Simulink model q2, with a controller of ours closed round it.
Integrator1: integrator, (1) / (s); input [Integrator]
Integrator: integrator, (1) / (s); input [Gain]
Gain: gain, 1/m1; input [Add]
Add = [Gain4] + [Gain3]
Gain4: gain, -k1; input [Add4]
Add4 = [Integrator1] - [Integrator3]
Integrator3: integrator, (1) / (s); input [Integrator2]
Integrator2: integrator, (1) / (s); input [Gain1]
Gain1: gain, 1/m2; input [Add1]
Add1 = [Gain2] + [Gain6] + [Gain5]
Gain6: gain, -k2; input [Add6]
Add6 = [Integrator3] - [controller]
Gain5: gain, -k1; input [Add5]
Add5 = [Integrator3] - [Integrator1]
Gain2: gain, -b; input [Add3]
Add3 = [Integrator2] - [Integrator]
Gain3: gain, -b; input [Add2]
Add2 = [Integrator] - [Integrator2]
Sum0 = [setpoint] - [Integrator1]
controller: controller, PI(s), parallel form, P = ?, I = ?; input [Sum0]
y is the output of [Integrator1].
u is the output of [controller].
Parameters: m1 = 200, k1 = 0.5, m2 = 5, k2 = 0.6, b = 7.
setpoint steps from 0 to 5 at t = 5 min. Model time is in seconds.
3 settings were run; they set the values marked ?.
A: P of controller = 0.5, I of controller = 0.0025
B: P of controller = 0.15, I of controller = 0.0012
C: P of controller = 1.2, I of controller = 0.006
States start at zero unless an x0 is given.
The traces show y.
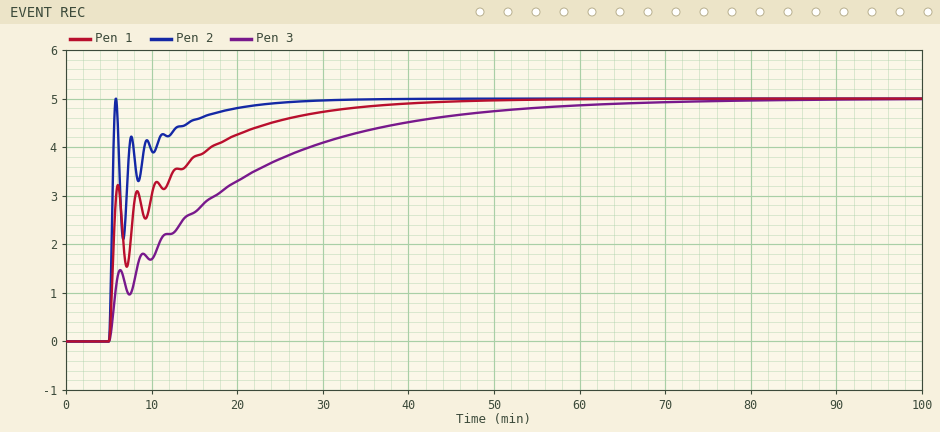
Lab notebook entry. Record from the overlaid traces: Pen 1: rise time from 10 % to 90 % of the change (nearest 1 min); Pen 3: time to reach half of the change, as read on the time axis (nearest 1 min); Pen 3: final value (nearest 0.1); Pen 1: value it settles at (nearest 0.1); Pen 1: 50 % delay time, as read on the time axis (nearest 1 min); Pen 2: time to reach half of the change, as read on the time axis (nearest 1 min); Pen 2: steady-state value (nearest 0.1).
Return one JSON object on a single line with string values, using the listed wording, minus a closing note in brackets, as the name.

{"Pen 1: rise time from 10 % to 90 % of the change": "19 min", "Pen 3: time to reach half of the change, as read on the time axis": "14 min", "Pen 3: final value": "5.0", "Pen 1: value it settles at": "5.0", "Pen 1: 50 % delay time, as read on the time axis": "6 min", "Pen 2: time to reach half of the change, as read on the time axis": "5 min", "Pen 2: steady-state value": "5.0"}
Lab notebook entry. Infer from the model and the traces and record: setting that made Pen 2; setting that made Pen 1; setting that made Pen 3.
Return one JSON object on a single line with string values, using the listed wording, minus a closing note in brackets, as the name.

{"setting that made Pen 2": "C", "setting that made Pen 1": "A", "setting that made Pen 3": "B"}
